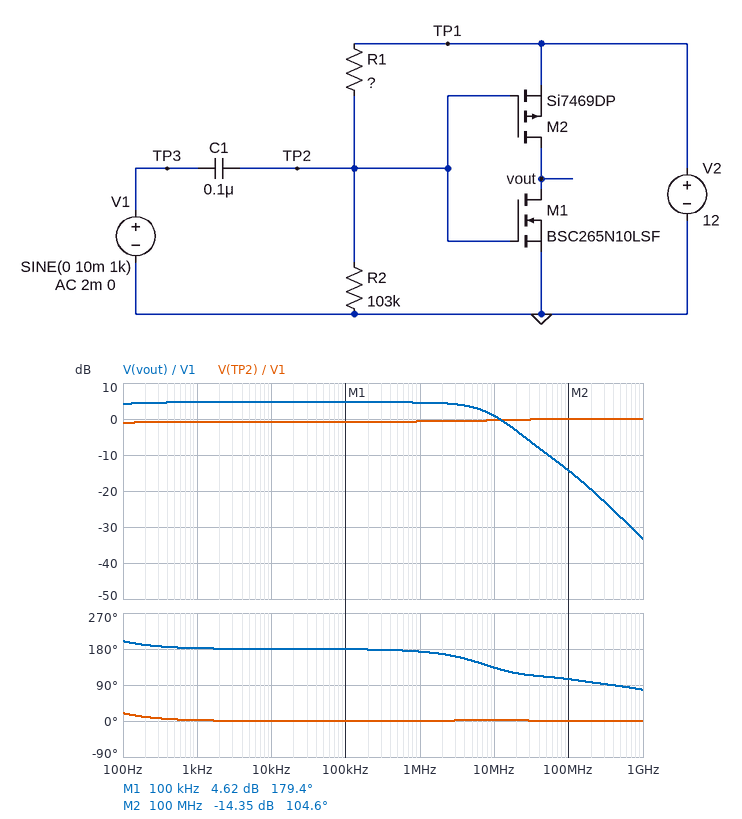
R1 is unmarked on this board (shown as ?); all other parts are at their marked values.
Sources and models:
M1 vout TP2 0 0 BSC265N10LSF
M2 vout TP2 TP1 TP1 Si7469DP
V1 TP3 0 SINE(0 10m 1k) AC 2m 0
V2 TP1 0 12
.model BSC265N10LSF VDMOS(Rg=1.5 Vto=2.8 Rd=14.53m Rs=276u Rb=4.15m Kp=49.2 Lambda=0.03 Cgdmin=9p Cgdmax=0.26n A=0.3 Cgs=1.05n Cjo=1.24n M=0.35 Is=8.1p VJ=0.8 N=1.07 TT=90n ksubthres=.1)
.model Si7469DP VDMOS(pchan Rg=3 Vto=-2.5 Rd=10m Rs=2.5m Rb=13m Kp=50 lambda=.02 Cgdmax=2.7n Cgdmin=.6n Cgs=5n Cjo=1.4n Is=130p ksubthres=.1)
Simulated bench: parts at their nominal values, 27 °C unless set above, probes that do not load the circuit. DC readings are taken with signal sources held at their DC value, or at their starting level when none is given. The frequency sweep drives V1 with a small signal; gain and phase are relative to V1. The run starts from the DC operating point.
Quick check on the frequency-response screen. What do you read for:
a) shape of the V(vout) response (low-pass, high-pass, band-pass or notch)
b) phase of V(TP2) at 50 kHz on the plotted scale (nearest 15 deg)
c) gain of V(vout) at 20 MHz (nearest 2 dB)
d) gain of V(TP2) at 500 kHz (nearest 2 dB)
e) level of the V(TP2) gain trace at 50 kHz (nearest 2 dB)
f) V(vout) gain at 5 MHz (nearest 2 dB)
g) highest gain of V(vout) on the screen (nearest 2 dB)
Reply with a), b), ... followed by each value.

a) low-pass
b) 0 deg
c) -4 dB
d) 0 dB
e) 0 dB
f) 4 dB
g) 4 dB
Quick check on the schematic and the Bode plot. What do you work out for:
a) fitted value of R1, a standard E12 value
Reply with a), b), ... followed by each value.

a) 68 kΩ
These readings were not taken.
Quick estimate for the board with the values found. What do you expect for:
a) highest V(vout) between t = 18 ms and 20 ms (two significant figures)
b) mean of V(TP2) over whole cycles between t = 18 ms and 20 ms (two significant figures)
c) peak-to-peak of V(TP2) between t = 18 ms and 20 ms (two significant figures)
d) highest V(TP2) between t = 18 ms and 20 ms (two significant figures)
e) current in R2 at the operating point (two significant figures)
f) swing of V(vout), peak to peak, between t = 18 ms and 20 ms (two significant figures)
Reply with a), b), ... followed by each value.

a) 2.3 V
b) 7.2 V
c) 18 mV
d) 7.2 V
e) 70 µA
f) 34 mV
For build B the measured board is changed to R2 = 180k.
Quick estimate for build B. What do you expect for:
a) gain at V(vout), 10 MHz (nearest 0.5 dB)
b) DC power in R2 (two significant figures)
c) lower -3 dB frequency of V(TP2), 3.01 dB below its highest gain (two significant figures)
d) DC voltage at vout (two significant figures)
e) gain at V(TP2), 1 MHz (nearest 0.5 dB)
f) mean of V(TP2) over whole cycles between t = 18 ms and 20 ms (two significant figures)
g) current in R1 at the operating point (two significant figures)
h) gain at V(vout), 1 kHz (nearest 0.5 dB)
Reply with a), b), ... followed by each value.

a) -6.5 dB
b) 420 µW
c) 35 Hz
d) 310 mV
e) -0.5 dB
f) 8.7 V
g) 48 µA
h) -3.0 dB
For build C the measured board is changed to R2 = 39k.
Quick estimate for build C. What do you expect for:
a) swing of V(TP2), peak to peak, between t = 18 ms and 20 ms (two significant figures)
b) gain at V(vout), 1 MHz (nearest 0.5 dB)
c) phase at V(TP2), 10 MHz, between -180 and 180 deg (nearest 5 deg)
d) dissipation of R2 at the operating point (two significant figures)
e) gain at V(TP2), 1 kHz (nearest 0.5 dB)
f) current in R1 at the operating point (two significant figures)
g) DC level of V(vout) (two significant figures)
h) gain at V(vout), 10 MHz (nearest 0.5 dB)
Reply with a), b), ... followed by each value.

a) 18 mV
b) 3.0 dB
c) 5 deg
d) 490 µW
e) -1.0 dB
f) 110 µA
g) 11 V
h) 3.5 dB
